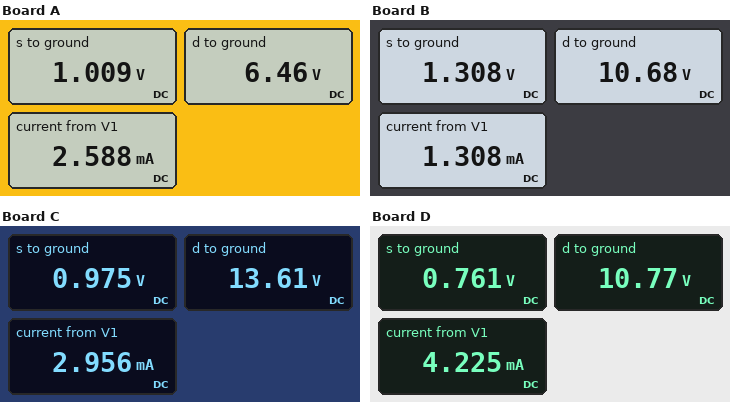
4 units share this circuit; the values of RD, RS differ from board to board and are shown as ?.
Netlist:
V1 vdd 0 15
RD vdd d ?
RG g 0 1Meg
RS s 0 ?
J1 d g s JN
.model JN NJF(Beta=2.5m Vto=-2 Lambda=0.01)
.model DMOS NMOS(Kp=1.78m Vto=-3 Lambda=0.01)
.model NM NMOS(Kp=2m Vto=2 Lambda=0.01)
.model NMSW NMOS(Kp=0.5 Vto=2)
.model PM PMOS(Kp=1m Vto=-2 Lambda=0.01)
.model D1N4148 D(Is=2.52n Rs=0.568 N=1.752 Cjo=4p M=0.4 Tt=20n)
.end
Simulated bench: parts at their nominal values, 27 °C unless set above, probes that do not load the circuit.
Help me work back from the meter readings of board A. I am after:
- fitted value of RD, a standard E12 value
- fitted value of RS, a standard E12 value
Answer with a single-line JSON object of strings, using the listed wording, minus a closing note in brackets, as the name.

{"fitted value of RD, a standard E12 value": "3.3 kΩ", "fitted value of RS, a standard E12 value": "390 Ω"}
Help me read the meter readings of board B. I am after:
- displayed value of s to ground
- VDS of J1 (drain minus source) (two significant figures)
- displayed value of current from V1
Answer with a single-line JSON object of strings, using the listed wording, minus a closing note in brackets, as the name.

{"displayed value of s to ground": "1.308 V", "VDS of J1 (drain minus source)": "9.4 V", "displayed value of current from V1": "1.308 mA"}
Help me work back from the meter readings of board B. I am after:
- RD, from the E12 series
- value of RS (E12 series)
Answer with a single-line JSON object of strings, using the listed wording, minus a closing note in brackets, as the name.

{"RD, from the E12 series": "3.3 kΩ", "value of RS": "1 kΩ"}
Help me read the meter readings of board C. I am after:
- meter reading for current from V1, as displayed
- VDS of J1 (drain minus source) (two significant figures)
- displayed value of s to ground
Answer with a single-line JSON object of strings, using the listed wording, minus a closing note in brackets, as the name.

{"meter reading for current from V1, as displayed": "2.956 mA", "VDS of J1 (drain minus source)": "13 V", "displayed value of s to ground": "0.975 V"}
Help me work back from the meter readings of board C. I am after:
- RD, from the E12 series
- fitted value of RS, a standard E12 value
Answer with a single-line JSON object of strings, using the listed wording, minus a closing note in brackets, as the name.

{"RD, from the E12 series": "470 Ω", "fitted value of RS, a standard E12 value": "330 Ω"}
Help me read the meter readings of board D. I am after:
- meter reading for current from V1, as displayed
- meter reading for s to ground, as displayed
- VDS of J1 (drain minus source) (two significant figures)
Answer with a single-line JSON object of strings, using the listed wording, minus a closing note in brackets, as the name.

{"meter reading for current from V1, as displayed": "4.225 mA", "meter reading for s to ground, as displayed": "0.761 V", "VDS of J1 (drain minus source)": "10 V"}
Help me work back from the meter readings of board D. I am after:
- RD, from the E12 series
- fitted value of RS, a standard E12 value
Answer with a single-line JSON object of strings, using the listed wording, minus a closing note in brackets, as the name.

{"RD, from the E12 series": "1 kΩ", "fitted value of RS, a standard E12 value": "180 Ω"}
